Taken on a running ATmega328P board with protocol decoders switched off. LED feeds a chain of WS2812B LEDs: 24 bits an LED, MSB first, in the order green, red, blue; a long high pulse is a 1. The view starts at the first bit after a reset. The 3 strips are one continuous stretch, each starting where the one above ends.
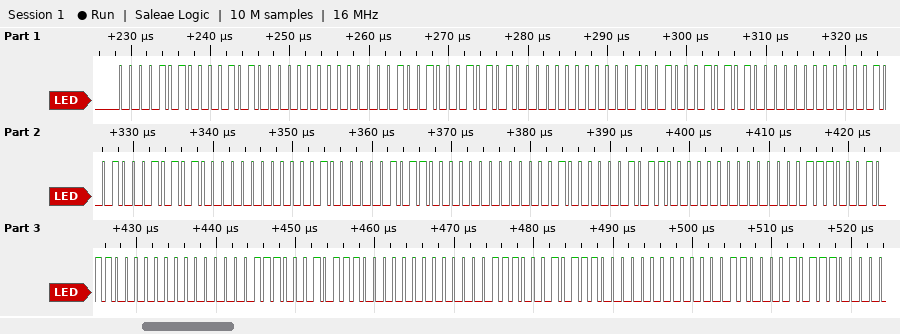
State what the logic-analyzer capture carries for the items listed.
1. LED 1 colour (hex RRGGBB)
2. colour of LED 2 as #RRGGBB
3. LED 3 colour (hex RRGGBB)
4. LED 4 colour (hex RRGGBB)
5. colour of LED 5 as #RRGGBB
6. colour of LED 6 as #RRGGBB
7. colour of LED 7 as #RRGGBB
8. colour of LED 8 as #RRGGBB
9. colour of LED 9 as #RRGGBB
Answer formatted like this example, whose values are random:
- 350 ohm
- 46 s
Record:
- #140A00
- #150900
- #150900
- #150900
- #160800
- #160800
- #160700
- #170700
- #170700
